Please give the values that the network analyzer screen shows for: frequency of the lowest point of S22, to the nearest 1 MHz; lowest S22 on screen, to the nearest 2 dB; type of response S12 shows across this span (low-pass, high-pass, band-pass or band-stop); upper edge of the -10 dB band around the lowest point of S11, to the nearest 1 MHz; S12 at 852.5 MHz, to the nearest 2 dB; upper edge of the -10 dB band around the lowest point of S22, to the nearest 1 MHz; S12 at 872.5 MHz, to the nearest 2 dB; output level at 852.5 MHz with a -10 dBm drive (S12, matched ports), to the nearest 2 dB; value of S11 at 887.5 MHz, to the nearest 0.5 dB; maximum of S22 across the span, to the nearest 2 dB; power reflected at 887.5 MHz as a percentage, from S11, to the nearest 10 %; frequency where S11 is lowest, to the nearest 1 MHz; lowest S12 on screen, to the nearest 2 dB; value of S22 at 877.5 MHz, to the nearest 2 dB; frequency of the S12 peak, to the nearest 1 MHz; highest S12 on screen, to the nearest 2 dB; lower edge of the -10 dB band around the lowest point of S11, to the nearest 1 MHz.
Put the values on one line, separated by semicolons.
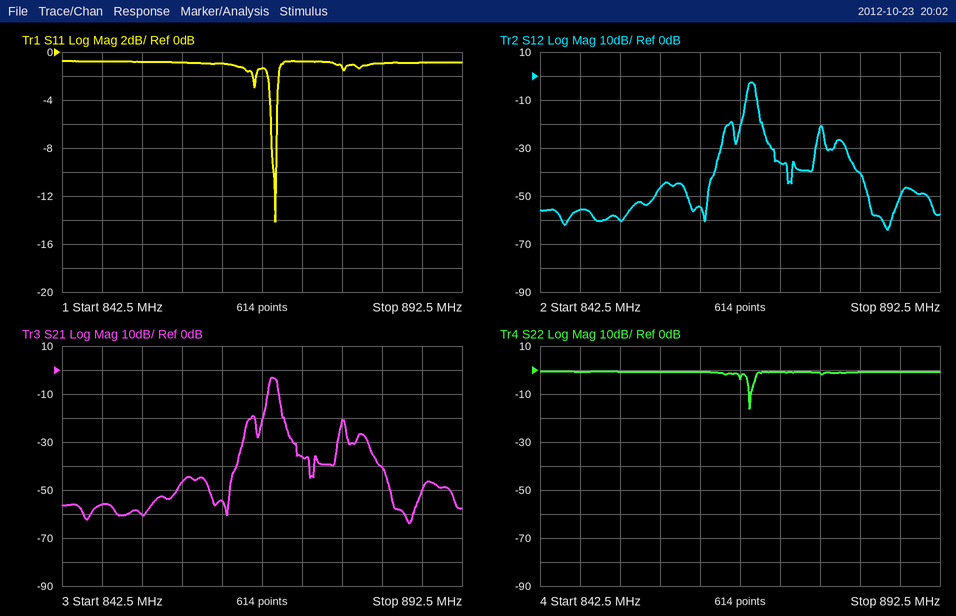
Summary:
869 MHz; -16 dB; band-pass; 869 MHz; -60 dB; 869 MHz; -36 dB; -70 dBm; -1.0 dB; 0 dB; 80 %; 869 MHz; -64 dB; -2 dB; 869 MHz; -2 dB; 869 MHz
